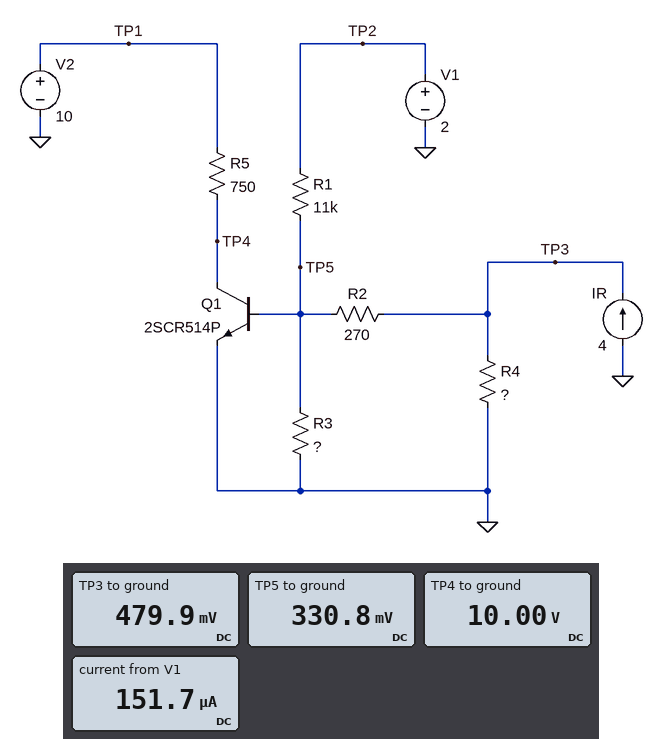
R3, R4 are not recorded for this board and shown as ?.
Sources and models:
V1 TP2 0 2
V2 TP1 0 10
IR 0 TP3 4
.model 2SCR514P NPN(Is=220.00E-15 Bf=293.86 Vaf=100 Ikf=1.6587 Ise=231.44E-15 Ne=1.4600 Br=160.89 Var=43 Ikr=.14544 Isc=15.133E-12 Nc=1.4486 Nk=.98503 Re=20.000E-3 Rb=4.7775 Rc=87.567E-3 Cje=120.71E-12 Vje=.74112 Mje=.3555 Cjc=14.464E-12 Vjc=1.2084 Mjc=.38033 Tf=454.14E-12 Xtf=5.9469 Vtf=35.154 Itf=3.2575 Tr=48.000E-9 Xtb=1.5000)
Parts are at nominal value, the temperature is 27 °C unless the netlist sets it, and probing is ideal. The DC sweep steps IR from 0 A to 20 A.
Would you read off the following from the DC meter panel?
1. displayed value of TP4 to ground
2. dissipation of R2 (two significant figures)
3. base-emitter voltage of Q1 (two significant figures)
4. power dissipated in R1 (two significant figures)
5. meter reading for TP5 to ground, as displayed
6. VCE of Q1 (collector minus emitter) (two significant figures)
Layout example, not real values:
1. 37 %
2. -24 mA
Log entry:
1. 10.00 V
2. 82 µW
3. 330 mV
4. 250 µW
5. 330.8 mV
6. 10 V
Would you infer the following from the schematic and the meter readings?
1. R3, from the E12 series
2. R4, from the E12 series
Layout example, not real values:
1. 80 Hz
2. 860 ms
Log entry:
1. 470 Ω
2. 0.12 Ω
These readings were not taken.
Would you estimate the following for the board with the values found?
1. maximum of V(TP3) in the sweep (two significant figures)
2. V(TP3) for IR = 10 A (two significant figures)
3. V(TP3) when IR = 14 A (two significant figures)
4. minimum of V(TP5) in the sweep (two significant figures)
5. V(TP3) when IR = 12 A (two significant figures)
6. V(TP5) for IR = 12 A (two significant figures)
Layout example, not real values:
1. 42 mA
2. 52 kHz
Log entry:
1. 2.4 V
2. 1.2 V
3. 1.7 V
4. 31 mV
5. 1.4 V
6. 690 mV
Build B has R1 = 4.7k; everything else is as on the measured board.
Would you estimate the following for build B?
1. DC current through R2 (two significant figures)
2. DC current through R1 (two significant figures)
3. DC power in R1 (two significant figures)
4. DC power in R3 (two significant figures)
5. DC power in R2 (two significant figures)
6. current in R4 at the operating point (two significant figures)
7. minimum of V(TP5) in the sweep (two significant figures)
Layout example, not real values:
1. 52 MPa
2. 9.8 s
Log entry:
1. 430 µA
2. 350 µA
3. 570 µW
4. 280 µW
5. 49 µW
6. 4.0 A
7. 70 mV
